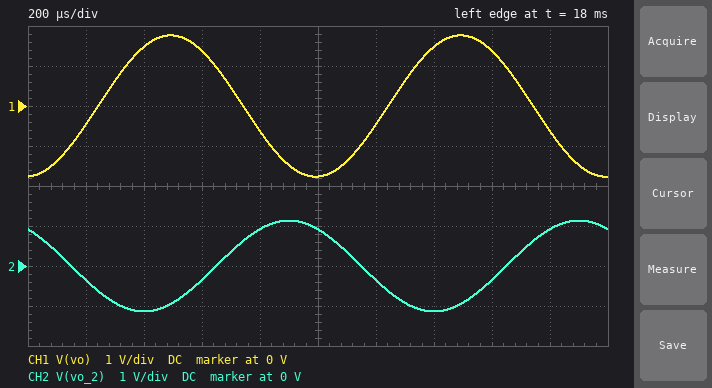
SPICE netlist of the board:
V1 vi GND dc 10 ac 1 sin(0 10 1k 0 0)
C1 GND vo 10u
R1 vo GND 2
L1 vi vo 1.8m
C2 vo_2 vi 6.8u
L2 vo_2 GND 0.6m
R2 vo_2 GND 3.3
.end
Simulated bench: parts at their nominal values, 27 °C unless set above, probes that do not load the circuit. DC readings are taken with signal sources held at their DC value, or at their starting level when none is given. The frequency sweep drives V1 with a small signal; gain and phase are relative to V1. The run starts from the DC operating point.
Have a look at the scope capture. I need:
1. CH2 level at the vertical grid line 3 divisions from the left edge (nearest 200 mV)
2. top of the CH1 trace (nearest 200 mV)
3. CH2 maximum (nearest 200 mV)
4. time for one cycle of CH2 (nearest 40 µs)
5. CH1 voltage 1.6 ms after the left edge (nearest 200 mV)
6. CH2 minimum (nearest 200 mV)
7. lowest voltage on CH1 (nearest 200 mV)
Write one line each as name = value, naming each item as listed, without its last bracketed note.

CH2 level at the vertical grid line 3 divisions from the left edge = -400 mV
top of the CH1 trace = 1.8 V
CH2 maximum = 1.2 V
time for one cycle of CH2 = 1.00 ms
CH1 voltage 1.6 ms after the left edge = 1.4 V
CH2 minimum = -1.2 V
lowest voltage on CH1 = -1.8 V
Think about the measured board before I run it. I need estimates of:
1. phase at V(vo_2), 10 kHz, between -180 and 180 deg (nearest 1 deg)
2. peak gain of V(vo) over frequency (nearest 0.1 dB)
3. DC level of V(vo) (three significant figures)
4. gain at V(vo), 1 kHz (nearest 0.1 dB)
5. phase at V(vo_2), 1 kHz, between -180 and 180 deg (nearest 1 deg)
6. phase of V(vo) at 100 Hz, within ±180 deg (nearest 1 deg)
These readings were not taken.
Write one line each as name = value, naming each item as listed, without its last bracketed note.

phase at V(vo_2), 10 kHz, between -180 and 180 deg = 37 deg
peak gain of V(vo) over frequency = 0 dB
DC level of V(vo) = 10.0 V
gain at V(vo), 1 kHz = -15.1 dB
phase at V(vo_2), 1 kHz, between -180 and 180 deg = 126 deg
phase of V(vo) at 100 Hz, within ±180 deg = -30 deg
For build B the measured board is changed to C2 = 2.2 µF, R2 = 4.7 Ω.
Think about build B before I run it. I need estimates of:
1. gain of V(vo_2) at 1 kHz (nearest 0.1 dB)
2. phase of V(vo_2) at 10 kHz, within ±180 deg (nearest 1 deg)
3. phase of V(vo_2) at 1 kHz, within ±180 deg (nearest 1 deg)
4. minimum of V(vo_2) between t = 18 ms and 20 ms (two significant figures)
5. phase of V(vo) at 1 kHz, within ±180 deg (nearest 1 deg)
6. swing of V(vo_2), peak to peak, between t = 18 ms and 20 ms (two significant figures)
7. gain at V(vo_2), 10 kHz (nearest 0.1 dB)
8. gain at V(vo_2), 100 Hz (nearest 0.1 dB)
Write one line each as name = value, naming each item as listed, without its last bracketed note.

gain of V(vo_2) at 1 kHz = -27.5 dB
phase of V(vo_2) at 10 kHz, within ±180 deg = 62 deg
phase of V(vo_2) at 1 kHz, within ±180 deg = 140 deg
minimum of V(vo_2) between t = 18 ms and 20 ms = -420 mV
phase of V(vo) at 1 kHz, within ±180 deg = -87 deg
swing of V(vo_2), peak to peak, between t = 18 ms and 20 ms = 840 mV
gain at V(vo_2), 10 kHz = -4.8 dB
gain at V(vo_2), 100 Hz = -65.7 dB
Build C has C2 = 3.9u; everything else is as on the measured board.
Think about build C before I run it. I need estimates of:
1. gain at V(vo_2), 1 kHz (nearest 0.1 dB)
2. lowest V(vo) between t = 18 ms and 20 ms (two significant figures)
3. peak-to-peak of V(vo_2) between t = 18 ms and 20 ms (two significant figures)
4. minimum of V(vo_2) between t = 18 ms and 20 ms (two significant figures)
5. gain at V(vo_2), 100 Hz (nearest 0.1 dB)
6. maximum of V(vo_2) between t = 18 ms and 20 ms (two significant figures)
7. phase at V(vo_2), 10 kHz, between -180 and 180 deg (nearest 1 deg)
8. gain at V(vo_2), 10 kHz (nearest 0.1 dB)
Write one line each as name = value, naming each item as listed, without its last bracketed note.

gain at V(vo_2), 1 kHz = -24.0 dB
lowest V(vo) between t = 18 ms and 20 ms = -1.8 V
peak-to-peak of V(vo_2) between t = 18 ms and 20 ms = 1.3 V
minimum of V(vo_2) between t = 18 ms and 20 ms = -630 mV
gain at V(vo_2), 100 Hz = -60.7 dB
maximum of V(vo_2) between t = 18 ms and 20 ms = 630 mV
phase at V(vo_2), 10 kHz, between -180 and 180 deg = 54 deg
gain at V(vo_2), 10 kHz = -3.7 dB
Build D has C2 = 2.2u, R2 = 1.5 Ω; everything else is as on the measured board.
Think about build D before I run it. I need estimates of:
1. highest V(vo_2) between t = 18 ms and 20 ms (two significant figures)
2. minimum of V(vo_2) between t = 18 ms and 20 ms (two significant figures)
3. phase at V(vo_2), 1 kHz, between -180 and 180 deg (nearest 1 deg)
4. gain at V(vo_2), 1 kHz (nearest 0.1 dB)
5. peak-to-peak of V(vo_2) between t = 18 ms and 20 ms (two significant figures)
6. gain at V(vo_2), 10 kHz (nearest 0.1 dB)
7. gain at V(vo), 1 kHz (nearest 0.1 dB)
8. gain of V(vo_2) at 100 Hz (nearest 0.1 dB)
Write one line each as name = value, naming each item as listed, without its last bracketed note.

highest V(vo_2) between t = 18 ms and 20 ms = 190 mV
minimum of V(vo_2) between t = 18 ms and 20 ms = -190 mV
phase at V(vo_2), 1 kHz, between -180 and 180 deg = 111 deg
gain at V(vo_2), 1 kHz = -34.2 dB
peak-to-peak of V(vo_2) between t = 18 ms and 20 ms = 390 mV
gain at V(vo_2), 10 kHz = -13.8 dB
gain at V(vo), 1 kHz = -15.1 dB
gain of V(vo_2) at 100 Hz = -65.9 dB
